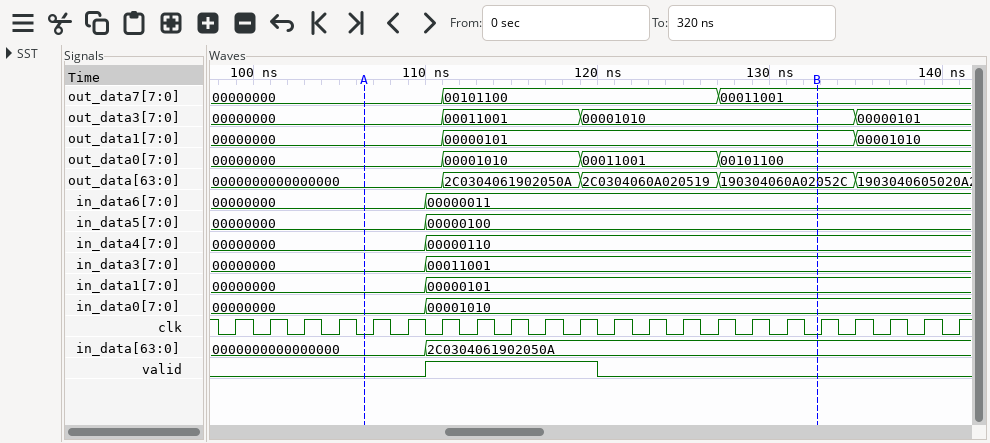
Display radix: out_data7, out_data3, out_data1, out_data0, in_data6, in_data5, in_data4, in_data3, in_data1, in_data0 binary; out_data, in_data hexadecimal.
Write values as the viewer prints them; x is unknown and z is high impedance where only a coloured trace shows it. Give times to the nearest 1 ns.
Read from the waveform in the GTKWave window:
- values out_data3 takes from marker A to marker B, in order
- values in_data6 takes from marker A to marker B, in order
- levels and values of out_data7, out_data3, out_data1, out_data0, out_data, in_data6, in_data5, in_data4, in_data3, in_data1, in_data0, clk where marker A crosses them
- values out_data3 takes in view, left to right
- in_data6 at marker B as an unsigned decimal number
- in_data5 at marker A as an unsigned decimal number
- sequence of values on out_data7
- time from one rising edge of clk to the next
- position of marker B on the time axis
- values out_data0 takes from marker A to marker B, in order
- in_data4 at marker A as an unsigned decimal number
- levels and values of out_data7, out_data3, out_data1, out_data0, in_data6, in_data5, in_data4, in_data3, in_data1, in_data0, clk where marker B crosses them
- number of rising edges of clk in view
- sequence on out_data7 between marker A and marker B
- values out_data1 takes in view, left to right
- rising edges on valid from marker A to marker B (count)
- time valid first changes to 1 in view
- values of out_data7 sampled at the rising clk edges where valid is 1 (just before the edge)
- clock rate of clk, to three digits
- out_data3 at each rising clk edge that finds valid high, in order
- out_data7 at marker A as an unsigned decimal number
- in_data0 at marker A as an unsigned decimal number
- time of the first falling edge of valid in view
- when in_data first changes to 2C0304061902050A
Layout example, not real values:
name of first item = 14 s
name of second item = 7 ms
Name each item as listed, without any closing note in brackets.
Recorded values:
values out_data3 takes from marker A to marker B, in order = 00000000, 00011001, 00001010
values in_data6 takes from marker A to marker B, in order = 00000000, 00000011
levels and values of out_data7, out_data3, out_data1, out_data0, out_data, in_data6, in_data5, in_data4, in_data3, in_data1, in_data0, clk where marker A crosses them = out_data7=00000000, out_data3=00000000, out_data1=00000000, out_data0=00000000, out_data=0000000000000000, in_data6=00000000, in_data5=00000000, in_data4=00000000, in_data3=00000000, in_data1=00000000, in_data0=00000000, clk=0
values out_data3 takes in view, left to right = 00000000, 00011001, 00001010, 00000101
in_data6 at marker B as an unsigned decimal number = 3
in_data5 at marker A as an unsigned decimal number = 0
sequence of values on out_data7 = 00000000, 00101100, 00011001
time from one rising edge of clk to the next = 2 ns
position of marker B on the time axis = 133 ns
values out_data0 takes from marker A to marker B, in order = 00000000, 00001010, 00011001, 00101100
in_data4 at marker A as an unsigned decimal number = 0
levels and values of out_data7, out_data3, out_data1, out_data0, in_data6, in_data5, in_data4, in_data3, in_data1, in_data0, clk where marker B crosses them = out_data7=00011001, out_data3=00001010, out_data1=00000101, out_data0=00101100, in_data6=00000011, in_data5=00000100, in_data4=00000110, in_data3=00011001, in_data1=00000101, in_data0=00001010, clk=0
number of rising edges of clk in view = 22
sequence on out_data7 between marker A and marker B = 00000000, 00101100, 00011001
values out_data1 takes in view, left to right = 00000000, 00000101, 00001010
rising edges on valid from marker A to marker B = 1
time valid first changes to 1 in view = 110 ns
values of out_data7 sampled at the rising clk edges where valid is 1 = 00000000, 00101100, 00101100, 00101100, 00101100
clock rate of clk, to three digits = 500 MHz
out_data3 at each rising clk edge that finds valid high, in order = 00000000, 00011001, 00011001, 00011001, 00011001
out_data7 at marker A as an unsigned decimal number = 0
in_data0 at marker A as an unsigned decimal number = 0
time of the first falling edge of valid in view = 120 ns
when in_data first changes to 2C0304061902050A = 110 ns
